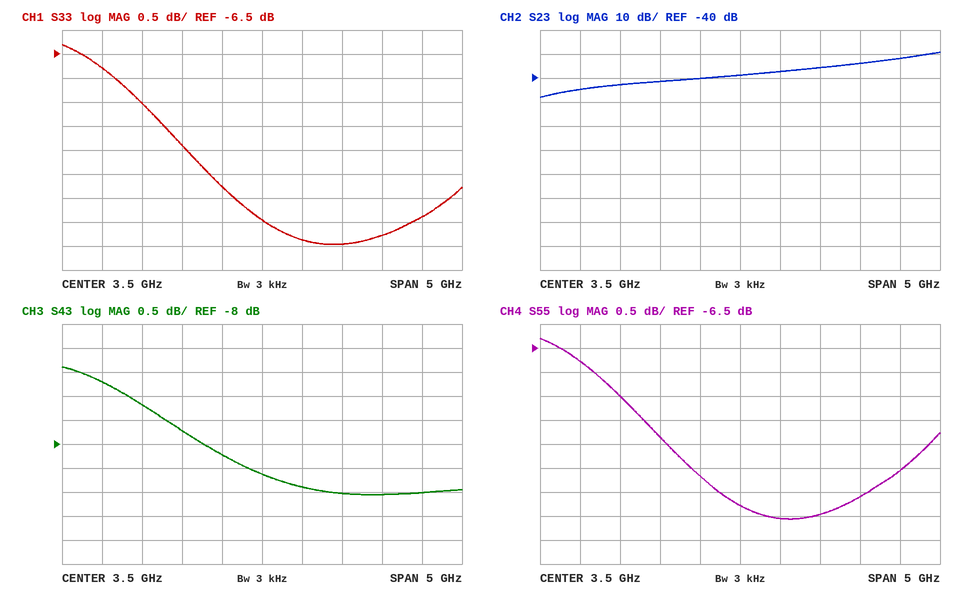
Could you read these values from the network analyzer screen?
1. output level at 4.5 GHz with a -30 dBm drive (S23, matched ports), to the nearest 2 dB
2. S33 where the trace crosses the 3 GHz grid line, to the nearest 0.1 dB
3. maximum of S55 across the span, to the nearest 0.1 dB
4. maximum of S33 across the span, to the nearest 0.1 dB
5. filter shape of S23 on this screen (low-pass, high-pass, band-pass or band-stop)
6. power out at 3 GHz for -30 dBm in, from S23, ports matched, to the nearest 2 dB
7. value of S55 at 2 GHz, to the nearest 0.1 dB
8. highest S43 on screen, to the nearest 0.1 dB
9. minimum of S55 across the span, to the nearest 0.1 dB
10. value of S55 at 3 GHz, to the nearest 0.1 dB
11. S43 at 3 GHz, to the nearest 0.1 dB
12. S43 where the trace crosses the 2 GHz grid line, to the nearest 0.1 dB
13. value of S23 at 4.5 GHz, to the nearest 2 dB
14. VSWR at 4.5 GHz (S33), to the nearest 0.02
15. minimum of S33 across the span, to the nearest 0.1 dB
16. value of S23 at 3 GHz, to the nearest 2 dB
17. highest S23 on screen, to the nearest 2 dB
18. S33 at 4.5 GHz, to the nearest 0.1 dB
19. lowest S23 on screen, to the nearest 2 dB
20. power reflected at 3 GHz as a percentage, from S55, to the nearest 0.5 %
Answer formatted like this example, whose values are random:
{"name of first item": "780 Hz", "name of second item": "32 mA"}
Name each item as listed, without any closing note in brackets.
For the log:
{"output level at 4.5 GHz with a -30 dBm drive (S23, matched ports), to the nearest 2 dB": "-66 dBm", "S33 where the trace crosses the 3 GHz grid line, to the nearest 0.1 dB": "-9.3 dB", "maximum of S55 across the span, to the nearest 0.1 dB": "-6.3 dB", "maximum of S33 across the span, to the nearest 0.1 dB": "-6.3 dB", "filter shape of S23 on this screen": "high-pass", "power out at 3 GHz for -30 dBm in, from S23, ports matched, to the nearest 2 dB": "-70 dBm", "value of S55 at 2 GHz, to the nearest 0.1 dB": "-7.5 dB", "highest S43 on screen, to the nearest 0.1 dB": "-6.4 dB", "minimum of S55 across the span, to the nearest 0.1 dB": "-10.1 dB", "value of S55 at 3 GHz, to the nearest 0.1 dB": "-9.2 dB", "S43 at 3 GHz, to the nearest 0.1 dB": "-8.2 dB", "S43 where the trace crosses the 2 GHz grid line, to the nearest 0.1 dB": "-7.2 dB", "value of S23 at 4.5 GHz, to the nearest 2 dB": "-36 dB", "VSWR at 4.5 GHz (S33), to the nearest 0.02": "1.86", "minimum of S33 across the span, to the nearest 0.1 dB": "-10.5 dB", "value of S23 at 3 GHz, to the nearest 2 dB": "-40 dB", "highest S23 on screen, to the nearest 2 dB": "-30 dB", "S33 at 4.5 GHz, to the nearest 0.1 dB": "-10.5 dB", "lowest S23 on screen, to the nearest 2 dB": "-48 dB", "power reflected at 3 GHz as a percentage, from S55, to the nearest 0.5 %": "12.0 %"}
